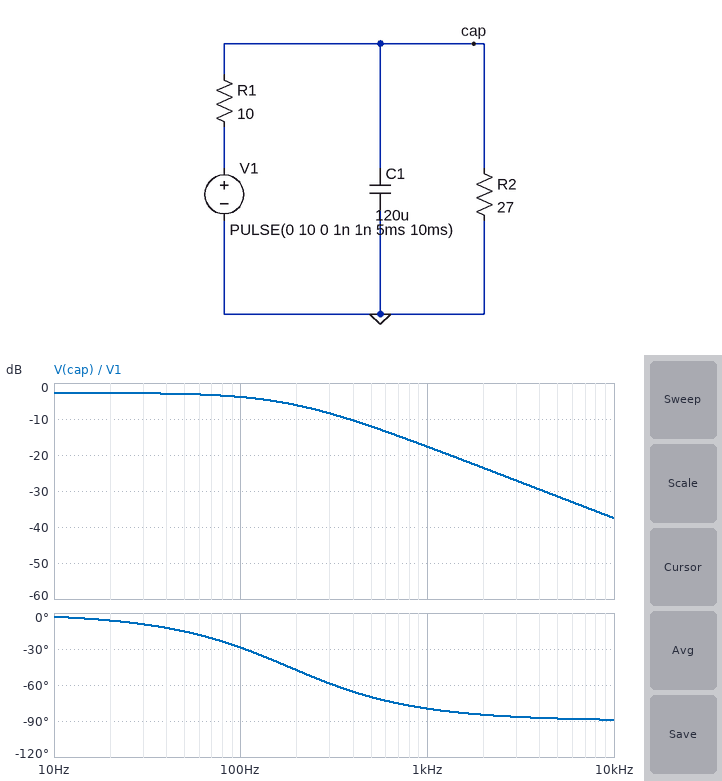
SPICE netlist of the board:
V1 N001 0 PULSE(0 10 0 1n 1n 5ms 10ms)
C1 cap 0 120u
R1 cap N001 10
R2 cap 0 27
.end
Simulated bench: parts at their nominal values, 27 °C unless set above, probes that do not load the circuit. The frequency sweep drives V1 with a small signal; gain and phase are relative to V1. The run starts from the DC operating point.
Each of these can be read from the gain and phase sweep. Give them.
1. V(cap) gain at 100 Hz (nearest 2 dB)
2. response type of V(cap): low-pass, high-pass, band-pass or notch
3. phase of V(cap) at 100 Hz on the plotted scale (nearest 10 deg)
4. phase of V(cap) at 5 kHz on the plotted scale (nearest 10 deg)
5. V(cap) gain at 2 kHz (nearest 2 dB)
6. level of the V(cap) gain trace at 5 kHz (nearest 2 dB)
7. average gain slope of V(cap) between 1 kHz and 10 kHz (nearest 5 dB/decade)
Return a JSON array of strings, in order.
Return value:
["-4 dB", "low-pass", "-30 deg", "-90 deg", "-24 dB", "-32 dB", "-20 dB/decade"]
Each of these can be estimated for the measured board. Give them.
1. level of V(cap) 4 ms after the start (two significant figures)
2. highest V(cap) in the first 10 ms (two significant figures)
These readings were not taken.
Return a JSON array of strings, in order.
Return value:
["7.2 V", "7.3 V"]
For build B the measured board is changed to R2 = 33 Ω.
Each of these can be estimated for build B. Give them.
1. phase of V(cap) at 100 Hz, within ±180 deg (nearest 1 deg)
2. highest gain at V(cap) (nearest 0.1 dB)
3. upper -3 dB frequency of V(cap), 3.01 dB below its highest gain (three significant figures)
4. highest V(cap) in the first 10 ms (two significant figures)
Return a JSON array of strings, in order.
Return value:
["-30 deg", "-2.3 dB", "173 Hz", "7.6 V"]
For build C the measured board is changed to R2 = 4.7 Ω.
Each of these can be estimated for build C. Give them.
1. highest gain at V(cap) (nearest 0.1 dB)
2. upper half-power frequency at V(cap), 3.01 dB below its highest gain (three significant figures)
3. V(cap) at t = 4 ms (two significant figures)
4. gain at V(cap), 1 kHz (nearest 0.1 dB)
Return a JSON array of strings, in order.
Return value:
["-9.9 dB", "415 Hz", "3.2 V", "-18.2 dB"]
